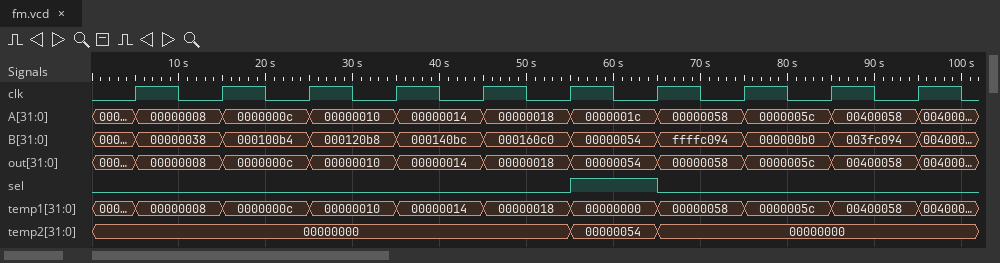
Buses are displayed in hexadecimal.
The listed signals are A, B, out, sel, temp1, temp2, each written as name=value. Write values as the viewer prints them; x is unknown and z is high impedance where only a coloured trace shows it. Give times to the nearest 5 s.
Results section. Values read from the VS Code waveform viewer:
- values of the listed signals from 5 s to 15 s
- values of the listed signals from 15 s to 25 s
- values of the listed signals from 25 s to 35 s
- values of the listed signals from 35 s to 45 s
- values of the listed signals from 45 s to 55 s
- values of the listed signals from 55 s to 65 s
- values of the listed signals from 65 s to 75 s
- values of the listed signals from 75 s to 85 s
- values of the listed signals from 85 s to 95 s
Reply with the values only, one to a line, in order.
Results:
A=00000008, B=00000038, out=00000008, sel=0, temp1=00000008, temp2=00000000
A=0000000c, B=000100b4, out=0000000c, sel=0, temp1=0000000c, temp2=00000000
A=00000010, B=000120b8, out=00000010, sel=0, temp1=00000010, temp2=00000000
A=00000014, B=000140bc, out=00000014, sel=0, temp1=00000014, temp2=00000000
A=00000018, B=000160c0, out=00000018, sel=0, temp1=00000018, temp2=00000000
A=0000001c, B=00000054, out=00000054, sel=1, temp1=00000000, temp2=00000054
A=00000058, B=ffffc094, out=00000058, sel=0, temp1=00000058, temp2=00000000
A=0000005c, B=000000b0, out=0000005c, sel=0, temp1=0000005c, temp2=00000000
A=00400058, B=003fc094, out=00400058, sel=0, temp1=00400058, temp2=00000000
